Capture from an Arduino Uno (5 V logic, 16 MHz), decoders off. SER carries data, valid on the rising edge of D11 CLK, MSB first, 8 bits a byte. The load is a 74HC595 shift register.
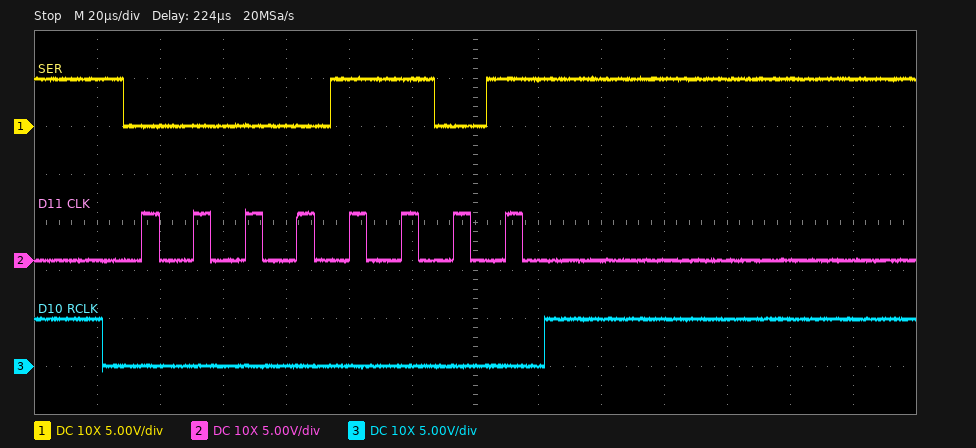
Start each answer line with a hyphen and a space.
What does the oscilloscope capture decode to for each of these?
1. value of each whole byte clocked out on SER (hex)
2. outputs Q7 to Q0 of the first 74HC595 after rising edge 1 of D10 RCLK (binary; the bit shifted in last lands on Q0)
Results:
- 0x0D
- 00001101
